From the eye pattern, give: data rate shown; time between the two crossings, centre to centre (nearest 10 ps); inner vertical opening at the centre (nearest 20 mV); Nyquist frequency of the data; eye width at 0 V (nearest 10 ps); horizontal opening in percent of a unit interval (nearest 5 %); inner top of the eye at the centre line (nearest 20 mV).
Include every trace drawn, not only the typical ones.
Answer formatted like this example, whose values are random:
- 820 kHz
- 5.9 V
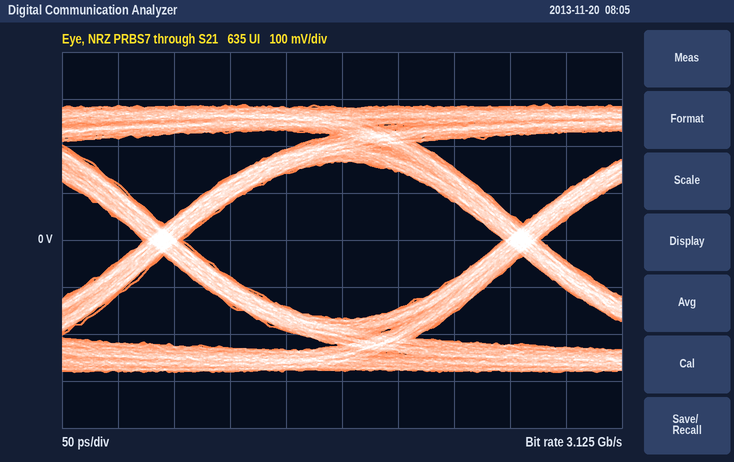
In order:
- 3.125 Gb/s
- 320 ps
- 340 mV
- 1.5625 GHz
- 290 ps
- 90 %
- 160 mV
